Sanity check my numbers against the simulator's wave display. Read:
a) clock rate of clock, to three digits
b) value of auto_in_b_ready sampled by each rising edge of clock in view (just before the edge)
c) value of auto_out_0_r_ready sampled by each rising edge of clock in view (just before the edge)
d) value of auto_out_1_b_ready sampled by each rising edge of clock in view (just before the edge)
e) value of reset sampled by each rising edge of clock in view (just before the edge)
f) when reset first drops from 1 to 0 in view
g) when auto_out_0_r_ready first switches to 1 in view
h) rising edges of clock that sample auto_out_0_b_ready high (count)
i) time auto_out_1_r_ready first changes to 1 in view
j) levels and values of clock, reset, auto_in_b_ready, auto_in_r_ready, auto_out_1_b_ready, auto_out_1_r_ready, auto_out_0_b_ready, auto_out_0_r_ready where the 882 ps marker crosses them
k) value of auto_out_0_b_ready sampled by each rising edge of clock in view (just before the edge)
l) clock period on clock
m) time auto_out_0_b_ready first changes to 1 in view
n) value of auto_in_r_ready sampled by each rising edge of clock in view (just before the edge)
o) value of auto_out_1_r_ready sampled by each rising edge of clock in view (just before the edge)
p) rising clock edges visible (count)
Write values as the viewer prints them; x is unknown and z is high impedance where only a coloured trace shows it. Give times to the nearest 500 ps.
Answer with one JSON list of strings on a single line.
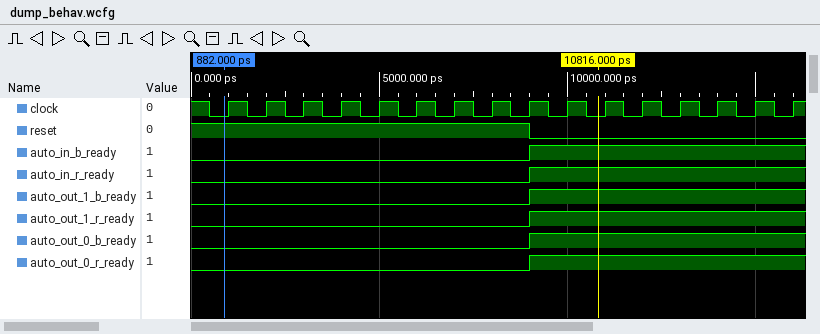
["1.00 GHz", "0 0 0 0 0 0 0 0 0 1 1 1 1 1 1 1", "0 0 0 0 0 0 0 0 0 1 1 1 1 1 1 1", "0 0 0 0 0 0 0 0 0 1 1 1 1 1 1 1", "1 1 1 1 1 1 1 1 1 0 0 0 0 0 0 0", "9000 ps", "9000 ps", "7", "9000 ps", "clock=0, reset=1, auto_in_b_ready=0, auto_in_r_ready=0, auto_out_1_b_ready=0, auto_out_1_r_ready=0, auto_out_0_b_ready=0, auto_out_0_r_ready=0", "0 0 0 0 0 0 0 0 0 1 1 1 1 1 1 1", "1000 ps", "9000 ps", "0 0 0 0 0 0 0 0 0 1 1 1 1 1 1 1", "0 0 0 0 0 0 0 0 0 1 1 1 1 1 1 1", "16"]
